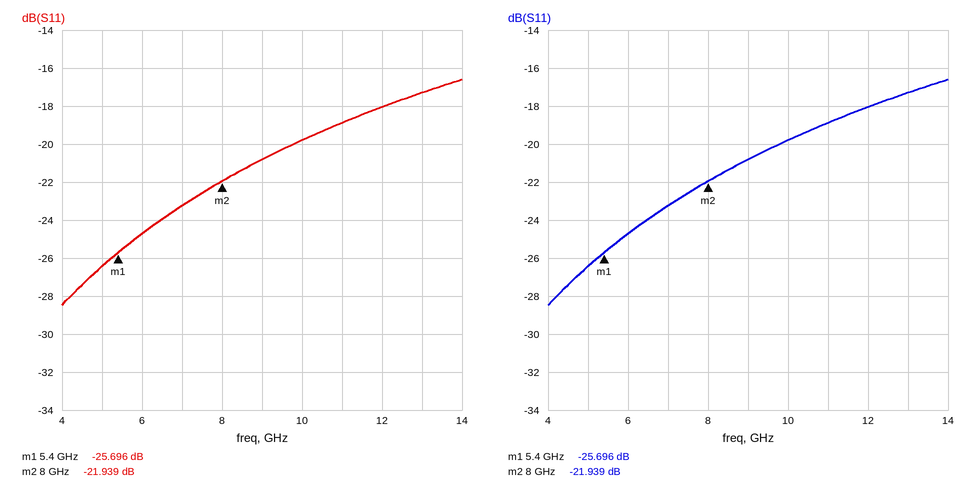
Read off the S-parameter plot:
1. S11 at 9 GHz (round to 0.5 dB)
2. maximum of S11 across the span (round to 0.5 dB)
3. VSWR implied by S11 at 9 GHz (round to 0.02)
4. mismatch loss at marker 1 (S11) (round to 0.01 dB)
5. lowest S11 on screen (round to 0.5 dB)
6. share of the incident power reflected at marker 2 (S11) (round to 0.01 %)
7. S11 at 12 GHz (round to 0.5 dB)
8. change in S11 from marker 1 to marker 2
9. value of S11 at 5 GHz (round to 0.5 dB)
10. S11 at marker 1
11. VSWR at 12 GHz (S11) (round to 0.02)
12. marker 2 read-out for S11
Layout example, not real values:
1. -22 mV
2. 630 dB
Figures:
1. -21.0 dB
2. -16.5 dB
3. 1.20
4. 0.01 dB
5. -28.5 dB
6. 0.64 %
7. -18.0 dB
8. 3.757 dB
9. -26.5 dB
10. -25.696 dB
11. 1.28
12. -21.939 dB
